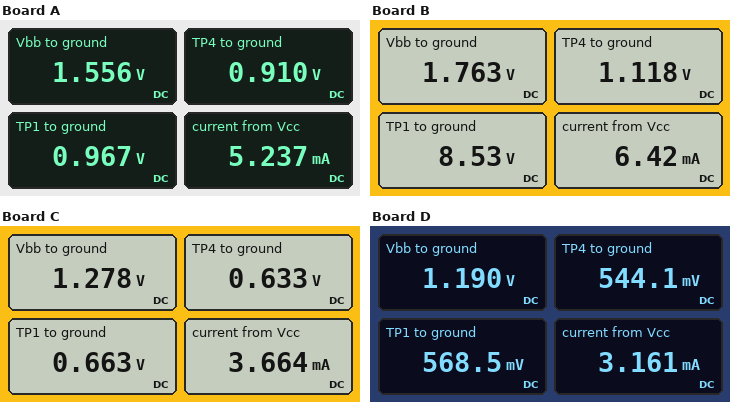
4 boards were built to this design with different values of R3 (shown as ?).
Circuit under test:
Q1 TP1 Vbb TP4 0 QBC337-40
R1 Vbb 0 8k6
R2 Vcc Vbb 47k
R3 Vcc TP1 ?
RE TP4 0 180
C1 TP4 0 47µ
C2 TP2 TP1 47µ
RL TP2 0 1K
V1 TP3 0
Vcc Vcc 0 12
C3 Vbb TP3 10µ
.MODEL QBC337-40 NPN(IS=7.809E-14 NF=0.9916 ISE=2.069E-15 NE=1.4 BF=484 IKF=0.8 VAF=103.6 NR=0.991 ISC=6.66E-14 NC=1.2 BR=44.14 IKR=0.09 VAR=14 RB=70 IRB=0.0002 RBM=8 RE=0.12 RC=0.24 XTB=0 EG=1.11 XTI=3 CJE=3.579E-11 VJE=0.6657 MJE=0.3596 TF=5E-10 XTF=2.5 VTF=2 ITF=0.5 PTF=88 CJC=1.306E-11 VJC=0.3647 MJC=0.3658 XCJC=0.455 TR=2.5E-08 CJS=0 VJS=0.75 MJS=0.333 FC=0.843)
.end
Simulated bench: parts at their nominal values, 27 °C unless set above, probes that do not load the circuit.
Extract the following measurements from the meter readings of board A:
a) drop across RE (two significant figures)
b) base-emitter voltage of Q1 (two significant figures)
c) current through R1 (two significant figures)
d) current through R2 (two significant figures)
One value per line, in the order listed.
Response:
910 mV
650 mV
180 µA
220 µA
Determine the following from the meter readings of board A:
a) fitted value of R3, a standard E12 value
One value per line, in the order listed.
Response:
2.2 kΩ
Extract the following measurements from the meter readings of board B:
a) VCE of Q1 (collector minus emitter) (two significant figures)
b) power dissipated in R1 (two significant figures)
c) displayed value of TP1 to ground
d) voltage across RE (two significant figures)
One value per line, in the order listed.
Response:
7.4 V
360 µW
8.53 V
1.1 V
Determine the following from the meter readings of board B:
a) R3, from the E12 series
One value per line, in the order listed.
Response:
560 Ω
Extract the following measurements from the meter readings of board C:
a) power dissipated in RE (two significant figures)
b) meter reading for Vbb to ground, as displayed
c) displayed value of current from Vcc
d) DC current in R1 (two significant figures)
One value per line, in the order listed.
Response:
2.2 mW
1.278 V
3.664 mA
150 µA
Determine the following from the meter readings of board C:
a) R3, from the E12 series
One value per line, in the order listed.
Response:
3.3 kΩ
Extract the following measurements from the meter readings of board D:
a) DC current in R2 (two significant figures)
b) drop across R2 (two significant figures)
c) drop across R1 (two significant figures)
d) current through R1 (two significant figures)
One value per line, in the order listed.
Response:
230 µA
11 V
1.2 V
140 µA
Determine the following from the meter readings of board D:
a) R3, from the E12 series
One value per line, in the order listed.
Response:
3.9 kΩ
